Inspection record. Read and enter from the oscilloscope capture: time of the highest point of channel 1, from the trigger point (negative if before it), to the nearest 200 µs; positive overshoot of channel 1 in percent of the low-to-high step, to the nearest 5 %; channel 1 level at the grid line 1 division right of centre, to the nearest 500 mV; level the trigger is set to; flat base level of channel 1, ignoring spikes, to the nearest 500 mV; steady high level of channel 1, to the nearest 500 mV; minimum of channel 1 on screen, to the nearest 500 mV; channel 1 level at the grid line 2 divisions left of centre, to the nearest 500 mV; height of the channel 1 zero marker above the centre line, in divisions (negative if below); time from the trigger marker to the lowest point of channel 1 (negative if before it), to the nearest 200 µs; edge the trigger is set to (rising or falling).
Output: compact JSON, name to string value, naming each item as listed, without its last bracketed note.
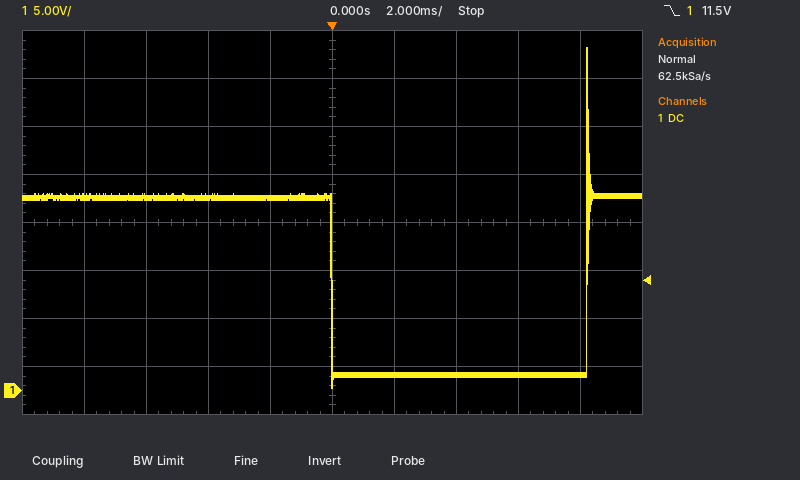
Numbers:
{"time of the highest point of channel 1, from the trigger point (negative if before it), to the nearest 200 µs": "+8.2 ms", "positive overshoot of channel 1 in percent of the low-to-high step, to the nearest 5 %": "85 %", "channel 1 level at the grid line 1 division right of centre, to the nearest 500 mV": "1.5 V", "level the trigger is set to": "11.5 V", "flat base level of channel 1, ignoring spikes, to the nearest 500 mV": "1.5 V", "steady high level of channel 1, to the nearest 500 mV": "20.0 V", "minimum of channel 1 on screen, to the nearest 500 mV": "500 mV", "channel 1 level at the grid line 2 divisions left of centre, to the nearest 500 mV": "20.0 V", "height of the channel 1 zero marker above the centre line, in divisions": "-3.5 div", "time from the trigger marker to the lowest point of channel 1 (negative if before it), to the nearest 200 µs": "0.0 ms", "edge the trigger is set to": "falling"}
